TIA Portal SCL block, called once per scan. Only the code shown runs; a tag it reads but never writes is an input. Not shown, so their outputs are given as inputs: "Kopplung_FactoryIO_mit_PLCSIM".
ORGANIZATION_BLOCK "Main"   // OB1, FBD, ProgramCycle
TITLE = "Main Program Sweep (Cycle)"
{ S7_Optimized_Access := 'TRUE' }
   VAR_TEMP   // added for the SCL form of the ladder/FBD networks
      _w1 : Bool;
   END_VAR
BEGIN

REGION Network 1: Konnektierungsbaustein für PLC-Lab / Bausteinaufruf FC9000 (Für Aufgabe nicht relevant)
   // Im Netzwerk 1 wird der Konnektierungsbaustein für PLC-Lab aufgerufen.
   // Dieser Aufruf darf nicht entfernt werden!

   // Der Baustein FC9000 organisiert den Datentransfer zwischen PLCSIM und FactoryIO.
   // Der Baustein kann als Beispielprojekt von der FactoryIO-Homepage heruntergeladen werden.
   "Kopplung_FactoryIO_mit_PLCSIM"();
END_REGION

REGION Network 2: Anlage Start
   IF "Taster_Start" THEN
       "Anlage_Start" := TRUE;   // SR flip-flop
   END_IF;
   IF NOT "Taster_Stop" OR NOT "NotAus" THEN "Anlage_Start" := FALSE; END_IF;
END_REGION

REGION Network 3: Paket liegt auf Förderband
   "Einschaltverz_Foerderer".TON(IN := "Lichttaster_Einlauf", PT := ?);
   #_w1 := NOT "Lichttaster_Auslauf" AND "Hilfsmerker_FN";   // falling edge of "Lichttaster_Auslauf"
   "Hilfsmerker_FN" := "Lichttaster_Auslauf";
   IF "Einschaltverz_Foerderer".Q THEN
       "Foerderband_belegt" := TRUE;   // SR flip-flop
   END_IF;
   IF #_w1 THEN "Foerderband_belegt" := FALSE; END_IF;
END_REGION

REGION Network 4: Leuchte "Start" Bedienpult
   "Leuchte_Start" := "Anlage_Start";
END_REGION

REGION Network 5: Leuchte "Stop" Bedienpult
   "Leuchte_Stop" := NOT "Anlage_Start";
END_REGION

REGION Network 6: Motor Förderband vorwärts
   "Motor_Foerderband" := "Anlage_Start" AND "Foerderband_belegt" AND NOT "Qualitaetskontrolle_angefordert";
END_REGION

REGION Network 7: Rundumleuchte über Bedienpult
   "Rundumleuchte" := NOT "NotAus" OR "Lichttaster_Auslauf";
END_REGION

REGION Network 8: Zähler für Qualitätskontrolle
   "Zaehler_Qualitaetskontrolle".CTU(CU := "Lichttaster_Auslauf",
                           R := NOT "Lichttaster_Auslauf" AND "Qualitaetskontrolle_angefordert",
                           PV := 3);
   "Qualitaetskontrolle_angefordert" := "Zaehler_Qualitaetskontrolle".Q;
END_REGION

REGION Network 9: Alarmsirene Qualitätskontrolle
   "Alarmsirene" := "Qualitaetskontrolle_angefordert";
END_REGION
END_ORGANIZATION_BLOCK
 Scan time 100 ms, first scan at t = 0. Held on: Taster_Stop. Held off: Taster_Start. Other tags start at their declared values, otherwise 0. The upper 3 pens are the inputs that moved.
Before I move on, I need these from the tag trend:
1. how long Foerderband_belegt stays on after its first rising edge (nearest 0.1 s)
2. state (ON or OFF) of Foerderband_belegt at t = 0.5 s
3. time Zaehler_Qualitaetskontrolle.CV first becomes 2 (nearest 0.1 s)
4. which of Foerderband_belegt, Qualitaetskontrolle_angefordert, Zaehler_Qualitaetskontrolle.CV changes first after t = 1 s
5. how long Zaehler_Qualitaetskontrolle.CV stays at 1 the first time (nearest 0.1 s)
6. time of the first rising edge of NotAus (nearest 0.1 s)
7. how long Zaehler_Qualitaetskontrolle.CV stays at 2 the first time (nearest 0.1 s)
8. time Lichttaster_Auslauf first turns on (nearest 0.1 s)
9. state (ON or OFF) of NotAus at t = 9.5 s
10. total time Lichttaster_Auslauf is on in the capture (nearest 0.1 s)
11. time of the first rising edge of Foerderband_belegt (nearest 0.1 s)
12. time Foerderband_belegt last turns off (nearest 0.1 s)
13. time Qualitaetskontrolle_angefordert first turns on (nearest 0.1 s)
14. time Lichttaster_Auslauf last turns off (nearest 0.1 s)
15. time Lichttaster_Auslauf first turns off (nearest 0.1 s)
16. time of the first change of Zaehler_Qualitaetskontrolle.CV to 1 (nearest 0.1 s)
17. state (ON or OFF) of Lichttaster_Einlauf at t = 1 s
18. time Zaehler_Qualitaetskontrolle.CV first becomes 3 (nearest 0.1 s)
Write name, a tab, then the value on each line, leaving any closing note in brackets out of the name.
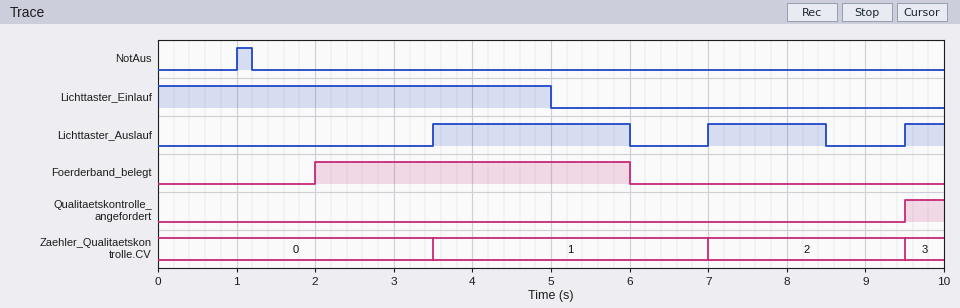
how long Foerderband_belegt stays on after its first rising edge	4.0 s
state (ON or OFF) of Foerderband_belegt at t = 0.5 s	OFF
time Zaehler_Qualitaetskontrolle.CV first becomes 2	7.0 s
which of Foerderband_belegt, Qualitaetskontrolle_angefordert, Zaehler_Qualitaetskontrolle.CV changes first after t = 1 s	Foerderband_belegt
how long Zaehler_Qualitaetskontrolle.CV stays at 1 the first time	3.5 s
time of the first rising edge of NotAus	1.0 s
how long Zaehler_Qualitaetskontrolle.CV stays at 2 the first time	2.5 s
time Lichttaster_Auslauf first turns on	3.5 s
state (ON or OFF) of NotAus at t = 9.5 s	OFF
total time Lichttaster_Auslauf is on in the capture	4.5 s
time of the first rising edge of Foerderband_belegt	2.0 s
time Foerderband_belegt last turns off	6.0 s
time Qualitaetskontrolle_angefordert first turns on	9.5 s
time Lichttaster_Auslauf last turns off	8.5 s
time Lichttaster_Auslauf first turns off	6.0 s
time of the first change of Zaehler_Qualitaetskontrolle.CV to 1	3.5 s
state (ON or OFF) of Lichttaster_Einlauf at t = 1 s	ON
time Zaehler_Qualitaetskontrolle.CV first becomes 3	9.5 s
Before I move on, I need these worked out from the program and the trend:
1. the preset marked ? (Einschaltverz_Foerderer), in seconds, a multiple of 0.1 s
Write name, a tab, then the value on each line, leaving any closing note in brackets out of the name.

the preset marked ? (Einschaltverz_Foerderer), in seconds, a multiple of 0.1 s	2.0 s
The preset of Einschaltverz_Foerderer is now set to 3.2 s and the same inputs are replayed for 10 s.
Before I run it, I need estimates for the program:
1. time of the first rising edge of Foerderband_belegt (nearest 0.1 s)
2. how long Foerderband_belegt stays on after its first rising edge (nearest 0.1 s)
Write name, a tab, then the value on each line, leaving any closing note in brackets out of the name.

time of the first rising edge of Foerderband_belegt	3.2 s
how long Foerderband_belegt stays on after its first rising edge	2.8 s
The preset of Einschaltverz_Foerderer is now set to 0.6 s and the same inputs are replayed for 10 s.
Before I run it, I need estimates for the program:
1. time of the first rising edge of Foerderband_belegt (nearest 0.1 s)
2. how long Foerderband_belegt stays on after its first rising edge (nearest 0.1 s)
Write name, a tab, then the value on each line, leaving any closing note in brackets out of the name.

time of the first rising edge of Foerderband_belegt	0.6 s
how long Foerderband_belegt stays on after its first rising edge	5.4 s
